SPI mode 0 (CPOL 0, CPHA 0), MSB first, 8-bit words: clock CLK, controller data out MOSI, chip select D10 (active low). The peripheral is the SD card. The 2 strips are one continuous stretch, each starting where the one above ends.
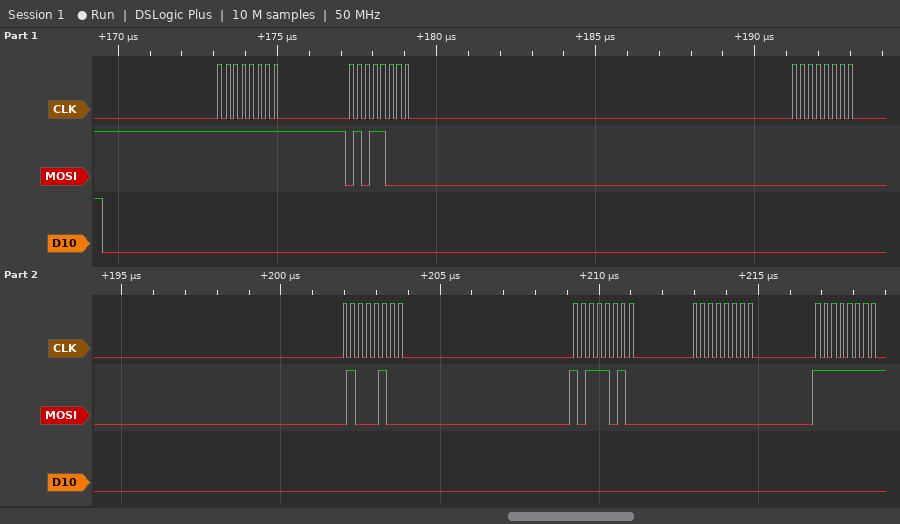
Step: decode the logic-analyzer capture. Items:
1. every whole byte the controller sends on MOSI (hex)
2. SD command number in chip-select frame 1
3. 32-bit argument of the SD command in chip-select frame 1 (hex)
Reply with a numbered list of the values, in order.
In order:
1. FF 58 00 44 BA 00 FF
2. CMD24
3. 0x0044BA00
